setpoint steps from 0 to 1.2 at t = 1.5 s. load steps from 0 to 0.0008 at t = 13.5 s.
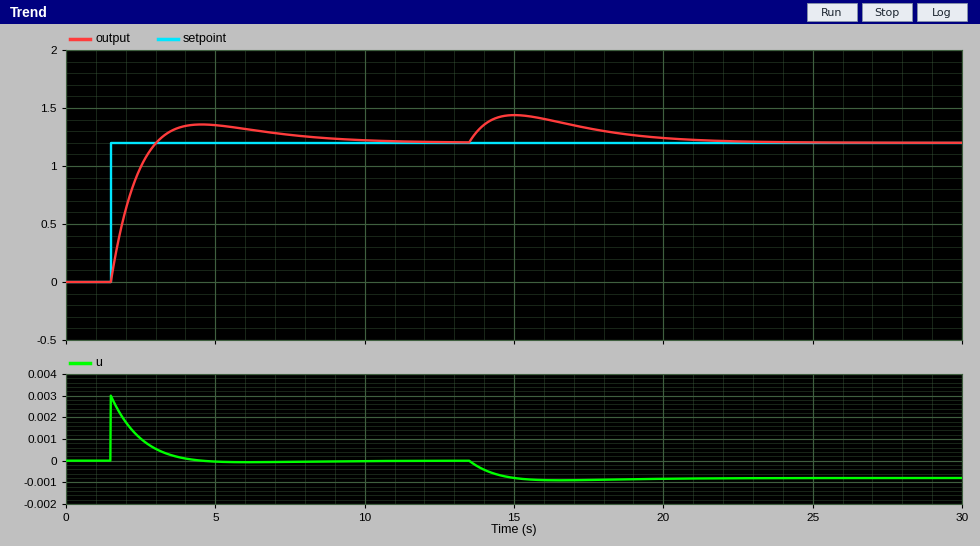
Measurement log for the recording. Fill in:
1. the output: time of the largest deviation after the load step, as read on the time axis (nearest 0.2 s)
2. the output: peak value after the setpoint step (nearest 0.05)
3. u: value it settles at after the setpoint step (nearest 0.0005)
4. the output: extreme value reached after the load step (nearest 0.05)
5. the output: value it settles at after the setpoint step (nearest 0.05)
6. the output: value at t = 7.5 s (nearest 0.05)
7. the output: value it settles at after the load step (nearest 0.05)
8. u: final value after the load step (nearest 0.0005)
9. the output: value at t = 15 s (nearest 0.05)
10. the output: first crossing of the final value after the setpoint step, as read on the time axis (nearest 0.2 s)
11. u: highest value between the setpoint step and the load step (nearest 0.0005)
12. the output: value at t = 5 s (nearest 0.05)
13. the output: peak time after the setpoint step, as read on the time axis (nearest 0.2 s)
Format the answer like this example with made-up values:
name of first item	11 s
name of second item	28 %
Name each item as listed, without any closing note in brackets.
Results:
the output: time of the largest deviation after the load step, as read on the time axis	15.0 s
the output: peak value after the setpoint step	1.35
u: value it settles at after the setpoint step	0.0000
the output: extreme value reached after the load step	1.45
the output: value it settles at after the setpoint step	1.20
the output: value at t = 7.5 s	1.25
the output: value it settles at after the load step	1.20
u: final value after the load step	-0.0010
the output: value at t = 15 s	1.45
the output: first crossing of the final value after the setpoint step, as read on the time axis	3.0 s
u: highest value between the setpoint step and the load step	0.0030
the output: value at t = 5 s	1.35
the output: peak time after the setpoint step, as read on the time axis	4.6 s
